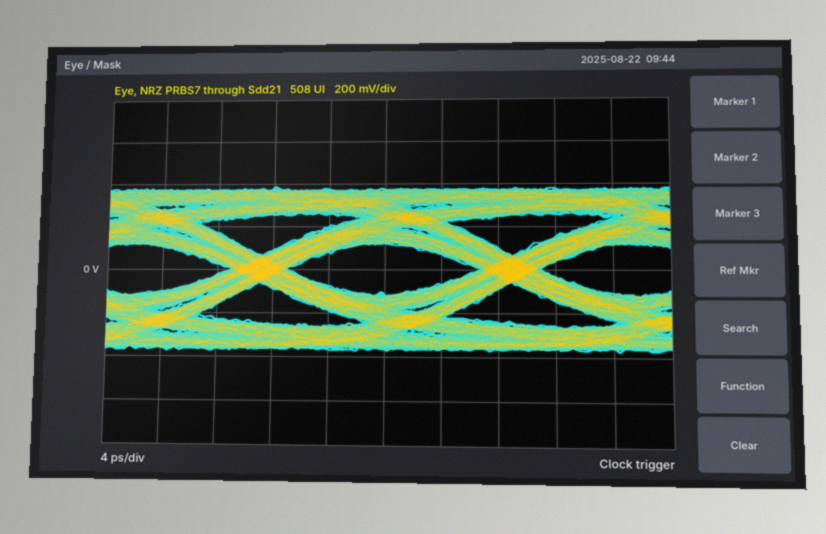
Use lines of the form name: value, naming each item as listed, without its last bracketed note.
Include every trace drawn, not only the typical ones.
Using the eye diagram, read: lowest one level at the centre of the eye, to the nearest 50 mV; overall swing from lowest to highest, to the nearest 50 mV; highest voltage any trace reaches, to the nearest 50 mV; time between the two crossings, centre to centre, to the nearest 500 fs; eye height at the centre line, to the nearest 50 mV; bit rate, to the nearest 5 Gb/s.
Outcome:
lowest one level at the centre of the eye, to the nearest 50 mV: 100 mV
overall swing from lowest to highest, to the nearest 50 mV: 750 mV
highest voltage any trace reaches, to the nearest 50 mV: 400 mV
time between the two crossings, centre to centre, to the nearest 500 fs: 18.0 ps
eye height at the centre line, to the nearest 50 mV: 250 mV
bit rate, to the nearest 5 Gb/s: 55 Gb/s
